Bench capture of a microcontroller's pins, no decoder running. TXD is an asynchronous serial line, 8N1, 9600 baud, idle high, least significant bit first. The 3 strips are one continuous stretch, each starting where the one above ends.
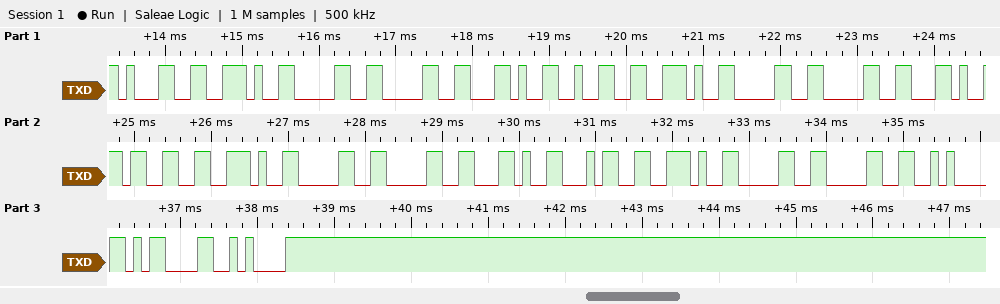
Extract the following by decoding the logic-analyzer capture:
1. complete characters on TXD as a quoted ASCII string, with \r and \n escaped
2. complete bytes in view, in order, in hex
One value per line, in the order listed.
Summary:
"1.00,2.00,3.00,4.00\n\r\n"
31 2E 30 30 2C 32 2E 30 30 2C 33 2E 30 30 2C 34 2E 30 30 0A 0D 0A
